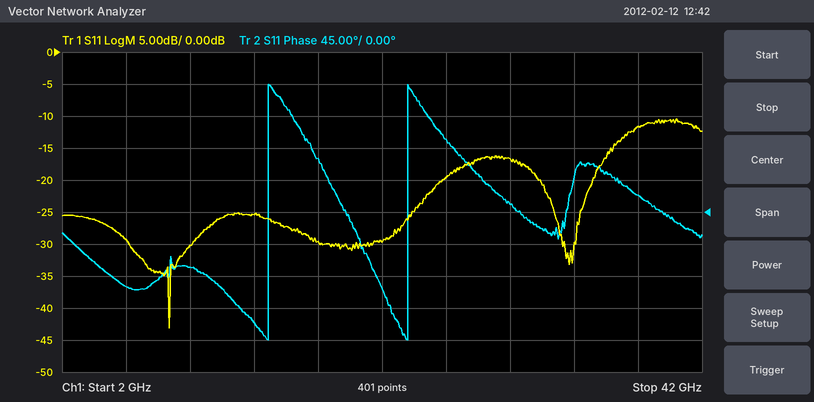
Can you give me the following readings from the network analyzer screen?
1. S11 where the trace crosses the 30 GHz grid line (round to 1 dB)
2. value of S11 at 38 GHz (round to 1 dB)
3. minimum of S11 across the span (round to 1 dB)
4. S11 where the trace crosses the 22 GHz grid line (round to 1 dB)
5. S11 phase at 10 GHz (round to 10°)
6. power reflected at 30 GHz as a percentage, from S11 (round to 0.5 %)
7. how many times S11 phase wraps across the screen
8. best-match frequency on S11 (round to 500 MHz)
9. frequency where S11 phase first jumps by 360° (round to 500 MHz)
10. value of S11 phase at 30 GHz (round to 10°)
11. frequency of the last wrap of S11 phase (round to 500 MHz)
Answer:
-17 dB
-12 dB
-43 dB
-30 dB
-80°
2.0 %
2
8.5 GHz
15.0 GHz
10°
23.5 GHz
